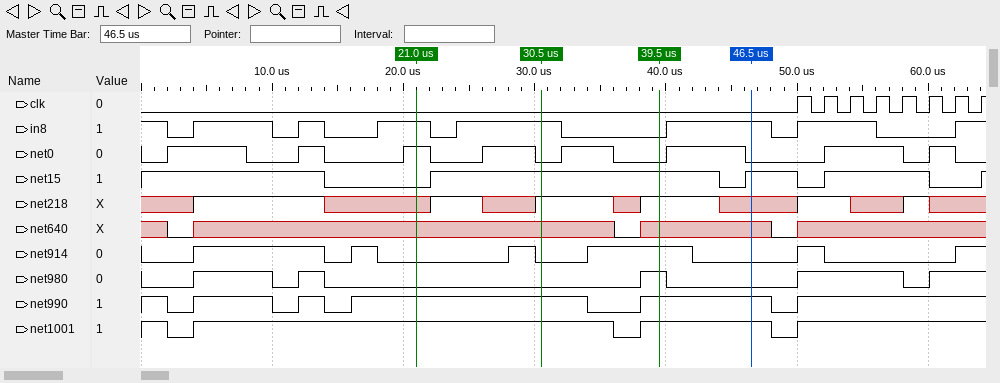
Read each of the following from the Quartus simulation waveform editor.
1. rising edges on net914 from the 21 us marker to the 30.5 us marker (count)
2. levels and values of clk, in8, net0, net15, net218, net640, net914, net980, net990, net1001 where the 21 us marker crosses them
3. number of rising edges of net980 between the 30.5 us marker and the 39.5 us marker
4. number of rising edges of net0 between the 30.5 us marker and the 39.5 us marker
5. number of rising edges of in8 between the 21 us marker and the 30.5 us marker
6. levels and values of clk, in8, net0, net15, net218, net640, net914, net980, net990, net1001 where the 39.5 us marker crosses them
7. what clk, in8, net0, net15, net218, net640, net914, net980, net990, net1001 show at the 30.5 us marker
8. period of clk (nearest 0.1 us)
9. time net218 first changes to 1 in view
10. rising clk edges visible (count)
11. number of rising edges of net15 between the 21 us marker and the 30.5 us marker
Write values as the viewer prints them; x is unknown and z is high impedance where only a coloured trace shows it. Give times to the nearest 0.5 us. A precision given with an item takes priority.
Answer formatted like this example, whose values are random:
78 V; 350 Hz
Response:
1; clk=0, in8=1, net0=1, net15=0, net218=x, net640=x, net914=0, net980=0, net990=1, net1001=1; 1; 1; 1; clk=0, in8=0, net0=0, net15=1, net218=1, net640=x, net914=1, net980=1, net990=1, net1001=1; clk=0, in8=1, net0=0, net15=1, net218=1, net640=x, net914=0, net980=0, net990=1, net1001=1; 2 us; 4 us; 8; 1
